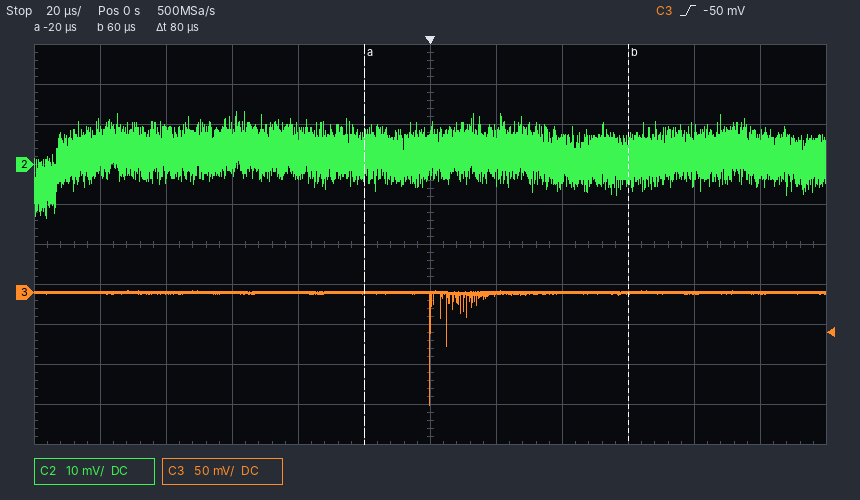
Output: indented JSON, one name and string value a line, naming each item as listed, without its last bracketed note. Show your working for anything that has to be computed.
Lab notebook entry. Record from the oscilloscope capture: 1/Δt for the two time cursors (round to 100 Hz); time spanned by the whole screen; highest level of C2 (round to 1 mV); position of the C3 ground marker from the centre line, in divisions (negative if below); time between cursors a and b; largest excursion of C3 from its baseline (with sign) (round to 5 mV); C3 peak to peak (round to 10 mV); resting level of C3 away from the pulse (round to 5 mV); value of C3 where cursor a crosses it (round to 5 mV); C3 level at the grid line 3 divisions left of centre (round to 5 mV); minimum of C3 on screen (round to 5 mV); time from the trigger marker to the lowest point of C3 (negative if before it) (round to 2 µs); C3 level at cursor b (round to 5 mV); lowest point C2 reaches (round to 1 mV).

{
  "1/Δt for the two time cursors": "1 / 80 µs ≈ 12.5 kHz",
  "time spanned by the whole screen": "240 µs",
  "highest level of C2": "13 mV",
  "position of the C3 ground marker from the centre line, in divisions": "-1.2 div",
  "time between cursors a and b": "80 µs",
  "largest excursion of C3 from its baseline (with sign)": "-140 mV − (0 mV) = -140 mV",
  "C3 peak to peak": "140 mV",
  "resting level of C3 away from the pulse": "0 mV",
  "value of C3 where cursor a crosses it": "0 mV",
  "C3 level at the grid line 3 divisions left of centre": "0 mV",
  "minimum of C3 on screen": "-140 mV",
  "time from the trigger marker to the lowest point of C3 (negative if before it)": "0 µs",
  "C3 level at cursor b": "0 mV",
  "lowest point C2 reaches": "-13 mV"
}
